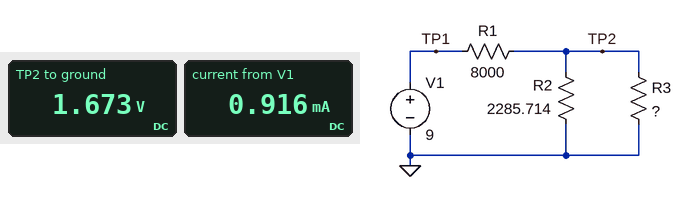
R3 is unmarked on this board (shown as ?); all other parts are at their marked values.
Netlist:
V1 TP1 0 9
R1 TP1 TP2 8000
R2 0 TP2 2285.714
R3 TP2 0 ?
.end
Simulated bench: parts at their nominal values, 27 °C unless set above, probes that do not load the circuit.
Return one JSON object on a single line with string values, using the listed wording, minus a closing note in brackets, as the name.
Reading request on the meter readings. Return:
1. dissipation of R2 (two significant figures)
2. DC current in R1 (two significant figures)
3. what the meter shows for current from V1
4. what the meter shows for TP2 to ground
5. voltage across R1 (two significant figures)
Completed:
{"dissipation of R2": "1.2 mW", "DC current in R1": "920 µA", "what the meter shows for current from V1": "0.916 mA", "what the meter shows for TP2 to ground": "1.673 V", "voltage across R1": "7.3 V"}
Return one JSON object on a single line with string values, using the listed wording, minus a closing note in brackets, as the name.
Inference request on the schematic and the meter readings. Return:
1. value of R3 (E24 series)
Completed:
{"value of R3": "9.1 kΩ"}
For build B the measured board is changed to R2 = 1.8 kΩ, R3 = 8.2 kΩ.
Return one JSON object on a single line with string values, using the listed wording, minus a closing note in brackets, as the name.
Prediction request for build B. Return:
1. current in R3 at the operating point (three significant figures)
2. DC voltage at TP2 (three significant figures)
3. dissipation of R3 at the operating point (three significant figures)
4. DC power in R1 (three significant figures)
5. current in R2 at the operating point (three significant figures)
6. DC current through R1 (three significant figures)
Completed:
{"current in R3 at the operating point": "171 µA", "DC voltage at TP2": "1.40 V", "dissipation of R3 at the operating point": "240 µW", "DC power in R1": "7.22 mW", "current in R2 at the operating point": "779 µA", "DC current through R1": "950 µA"}
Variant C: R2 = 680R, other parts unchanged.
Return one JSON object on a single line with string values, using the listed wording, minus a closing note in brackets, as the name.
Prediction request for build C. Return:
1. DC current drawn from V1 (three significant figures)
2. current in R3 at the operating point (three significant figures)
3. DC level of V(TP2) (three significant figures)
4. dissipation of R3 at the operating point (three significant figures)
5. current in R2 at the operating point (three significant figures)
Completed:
{"DC current drawn from V1": "1.04 mA", "current in R3 at the operating point": "72.5 µA", "DC level of V(TP2)": "660 mV", "dissipation of R3 at the operating point": "47.8 µW", "current in R2 at the operating point": "970 µA"}
